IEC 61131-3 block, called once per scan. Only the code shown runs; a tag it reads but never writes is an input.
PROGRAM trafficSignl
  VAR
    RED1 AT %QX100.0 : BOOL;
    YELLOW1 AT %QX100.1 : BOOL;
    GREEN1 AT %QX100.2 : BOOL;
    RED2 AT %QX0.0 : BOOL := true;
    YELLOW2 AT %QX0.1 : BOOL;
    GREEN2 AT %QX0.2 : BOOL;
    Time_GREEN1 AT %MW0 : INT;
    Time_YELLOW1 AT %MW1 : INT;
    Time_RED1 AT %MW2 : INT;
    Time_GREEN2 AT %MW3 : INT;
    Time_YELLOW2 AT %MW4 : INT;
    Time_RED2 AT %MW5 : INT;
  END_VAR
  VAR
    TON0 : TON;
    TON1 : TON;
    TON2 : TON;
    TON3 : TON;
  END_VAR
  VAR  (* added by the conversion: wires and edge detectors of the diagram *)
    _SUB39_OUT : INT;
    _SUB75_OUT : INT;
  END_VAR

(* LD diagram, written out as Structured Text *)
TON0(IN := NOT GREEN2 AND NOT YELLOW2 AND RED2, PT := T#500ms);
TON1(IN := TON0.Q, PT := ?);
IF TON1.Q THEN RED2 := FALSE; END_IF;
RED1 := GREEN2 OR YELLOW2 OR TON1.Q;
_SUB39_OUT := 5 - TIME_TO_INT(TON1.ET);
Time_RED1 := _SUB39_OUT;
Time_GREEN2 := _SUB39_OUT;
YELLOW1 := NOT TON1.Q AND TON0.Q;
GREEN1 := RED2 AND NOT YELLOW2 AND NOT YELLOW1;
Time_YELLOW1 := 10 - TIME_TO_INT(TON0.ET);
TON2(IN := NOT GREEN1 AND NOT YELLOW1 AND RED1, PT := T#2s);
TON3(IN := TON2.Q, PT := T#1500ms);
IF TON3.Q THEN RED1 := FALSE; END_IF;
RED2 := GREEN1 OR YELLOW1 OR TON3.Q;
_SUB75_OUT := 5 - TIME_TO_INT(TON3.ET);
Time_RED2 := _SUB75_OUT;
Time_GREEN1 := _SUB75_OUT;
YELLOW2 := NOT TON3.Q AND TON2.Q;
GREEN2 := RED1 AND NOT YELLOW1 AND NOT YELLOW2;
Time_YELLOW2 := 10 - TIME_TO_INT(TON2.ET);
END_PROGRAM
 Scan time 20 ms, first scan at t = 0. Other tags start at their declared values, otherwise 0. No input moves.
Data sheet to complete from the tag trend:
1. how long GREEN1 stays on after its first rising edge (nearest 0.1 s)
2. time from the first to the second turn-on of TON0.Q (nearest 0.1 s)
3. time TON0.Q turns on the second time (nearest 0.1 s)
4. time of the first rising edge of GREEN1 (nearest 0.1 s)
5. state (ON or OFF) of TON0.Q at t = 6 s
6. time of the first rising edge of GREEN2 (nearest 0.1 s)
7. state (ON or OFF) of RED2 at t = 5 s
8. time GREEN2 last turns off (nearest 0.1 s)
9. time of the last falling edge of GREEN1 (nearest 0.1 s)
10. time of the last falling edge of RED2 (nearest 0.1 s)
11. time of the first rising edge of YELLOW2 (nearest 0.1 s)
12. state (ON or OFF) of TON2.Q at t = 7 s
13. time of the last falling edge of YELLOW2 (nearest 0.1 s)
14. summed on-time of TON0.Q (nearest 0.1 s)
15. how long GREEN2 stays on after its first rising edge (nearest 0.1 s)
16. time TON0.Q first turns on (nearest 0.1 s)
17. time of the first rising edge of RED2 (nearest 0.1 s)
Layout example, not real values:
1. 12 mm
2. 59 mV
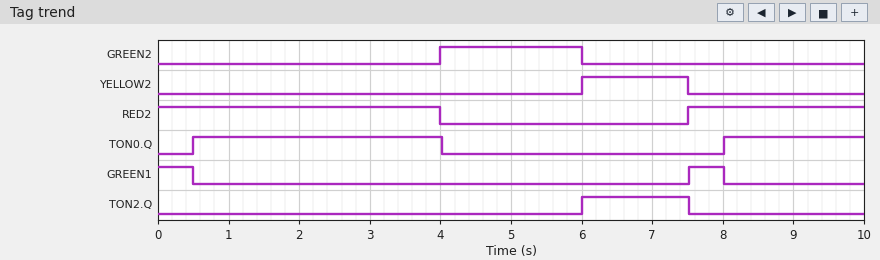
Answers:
1. 0.5 s
2. 7.5 s
3. 8.0 s
4. 7.5 s
5. OFF
6. 4.0 s
7. OFF
8. 6.0 s
9. 8.0 s
10. 4.0 s
11. 6.0 s
12. ON
13. 7.5 s
14. 5.5 s
15. 2.0 s
16. 0.5 s
17. 7.5 s
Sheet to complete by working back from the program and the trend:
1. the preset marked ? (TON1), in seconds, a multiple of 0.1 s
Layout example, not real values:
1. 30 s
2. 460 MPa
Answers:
1. 3.5 s
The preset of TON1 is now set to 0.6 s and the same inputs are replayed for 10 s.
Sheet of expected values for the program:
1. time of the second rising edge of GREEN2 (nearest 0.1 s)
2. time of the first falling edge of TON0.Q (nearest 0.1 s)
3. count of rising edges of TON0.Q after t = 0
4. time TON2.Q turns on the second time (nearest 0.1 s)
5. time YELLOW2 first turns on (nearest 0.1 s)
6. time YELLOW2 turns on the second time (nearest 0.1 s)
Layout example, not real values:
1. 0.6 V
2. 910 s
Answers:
1. 5.7 s
2. 1.1 s
3. 3
4. 7.7 s
5. 3.1 s
6. 7.7 s
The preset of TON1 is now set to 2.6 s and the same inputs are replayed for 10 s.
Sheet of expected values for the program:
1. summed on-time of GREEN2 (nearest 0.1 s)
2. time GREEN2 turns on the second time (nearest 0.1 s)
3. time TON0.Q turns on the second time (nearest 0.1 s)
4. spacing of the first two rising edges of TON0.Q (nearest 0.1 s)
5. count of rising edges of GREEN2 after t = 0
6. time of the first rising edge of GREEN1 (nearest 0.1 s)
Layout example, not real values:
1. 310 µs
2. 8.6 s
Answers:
1. 2.3 s
2. 9.7 s
3. 7.1 s
4. 6.6 s
5. 2
6. 6.6 s
